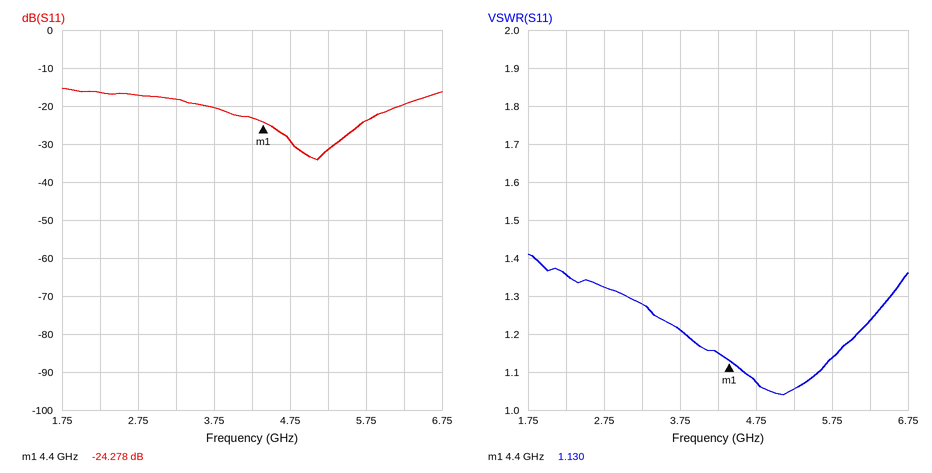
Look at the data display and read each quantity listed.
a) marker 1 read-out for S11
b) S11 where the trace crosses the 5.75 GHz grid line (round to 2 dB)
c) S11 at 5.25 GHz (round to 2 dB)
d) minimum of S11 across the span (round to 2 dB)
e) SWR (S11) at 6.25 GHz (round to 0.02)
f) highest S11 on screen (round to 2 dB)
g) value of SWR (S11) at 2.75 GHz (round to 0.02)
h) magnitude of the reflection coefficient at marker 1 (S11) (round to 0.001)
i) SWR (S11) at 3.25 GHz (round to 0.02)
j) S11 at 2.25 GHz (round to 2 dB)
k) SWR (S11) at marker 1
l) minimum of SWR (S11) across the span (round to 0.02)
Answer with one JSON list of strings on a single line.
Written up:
["-24.278 dB", "-24 dB", "-32 dB", "-34 dB", "1.24", "-16 dB", "1.32", "0.061", "1.28", "-16 dB", "1.130", "1.04"]
